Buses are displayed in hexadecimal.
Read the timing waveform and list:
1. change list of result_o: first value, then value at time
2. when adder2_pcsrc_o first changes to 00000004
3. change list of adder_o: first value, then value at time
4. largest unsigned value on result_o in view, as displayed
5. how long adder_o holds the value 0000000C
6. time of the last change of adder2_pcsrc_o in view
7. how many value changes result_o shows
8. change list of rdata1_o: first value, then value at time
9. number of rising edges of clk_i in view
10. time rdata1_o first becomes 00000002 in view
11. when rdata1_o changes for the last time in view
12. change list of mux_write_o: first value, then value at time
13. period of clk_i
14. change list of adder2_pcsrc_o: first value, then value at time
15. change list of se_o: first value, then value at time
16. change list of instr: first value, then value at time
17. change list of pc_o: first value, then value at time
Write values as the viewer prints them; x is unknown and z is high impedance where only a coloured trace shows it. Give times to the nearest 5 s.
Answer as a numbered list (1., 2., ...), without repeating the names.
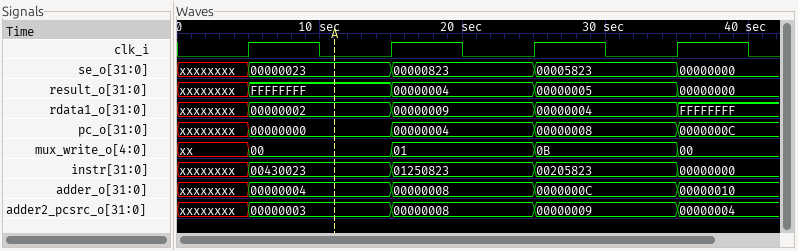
1. xxxxxxxx, FFFFFFFF at 5 s, 00000004 at 15 s, 00000005 at 25 s, 00000000 at 35 s
2. 35 s
3. xxxxxxxx, 00000004 at 5 s, 00000008 at 15 s, 0000000C at 25 s, 00000010 at 35 s
4. FFFFFFFF
5. 10 s
6. 35 s
7. 4
8. xxxxxxxx, 00000002 at 5 s, 00000009 at 15 s, 00000004 at 25 s, FFFFFFFF at 35 s
9. 4
10. 5 s
11. 35 s
12. xx, 00 at 5 s, 01 at 15 s, 0B at 25 s, 00 at 35 s
13. 10 s
14. xxxxxxxx, 00000003 at 5 s, 00000008 at 15 s, 00000009 at 25 s, 00000004 at 35 s
15. xxxxxxxx, 00000023 at 5 s, 00000823 at 15 s, 00005823 at 25 s, 00000000 at 35 s
16. xxxxxxxx, 00430023 at 5 s, 01250823 at 15 s, 00205823 at 25 s, 00000000 at 35 s
17. xxxxxxxx, 00000000 at 5 s, 00000004 at 15 s, 00000008 at 25 s, 0000000C at 35 s
